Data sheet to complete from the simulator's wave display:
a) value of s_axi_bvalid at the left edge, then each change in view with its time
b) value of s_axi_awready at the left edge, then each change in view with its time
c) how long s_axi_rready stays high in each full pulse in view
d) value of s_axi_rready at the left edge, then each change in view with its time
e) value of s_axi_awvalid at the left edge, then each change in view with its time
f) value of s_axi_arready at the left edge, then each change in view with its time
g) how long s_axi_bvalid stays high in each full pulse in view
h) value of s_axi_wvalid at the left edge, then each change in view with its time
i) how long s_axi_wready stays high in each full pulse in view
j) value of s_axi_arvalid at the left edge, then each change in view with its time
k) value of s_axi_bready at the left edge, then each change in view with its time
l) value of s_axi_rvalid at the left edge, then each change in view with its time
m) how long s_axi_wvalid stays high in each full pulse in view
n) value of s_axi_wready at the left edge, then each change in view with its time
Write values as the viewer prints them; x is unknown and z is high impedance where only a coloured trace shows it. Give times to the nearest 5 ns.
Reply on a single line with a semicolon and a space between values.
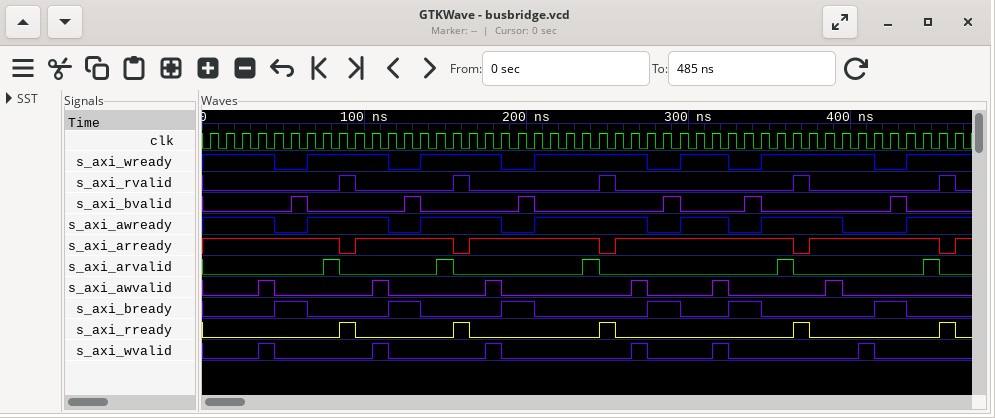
0, 1 at 55 ns, 0 at 65 ns, 1 at 125 ns, 0 at 135 ns, 1 at 195 ns, 0 at 205 ns, 1 at 285 ns, 0 at 295 ns, 1 at 335 ns, 0 at 345 ns, 1 at 425 ns, 0 at 435 ns; 1, 0 at 45 ns, 1 at 65 ns, 0 at 115 ns, 1 at 135 ns, 0 at 185 ns, 1 at 205 ns, 0 at 275 ns, 1 at 295 ns, 0 at 325 ns, 1 at 345 ns, 0 at 395 ns, 1 at 435 ns; 10 ns, 10 ns, 10 ns, 10 ns, 10 ns; 0, 1 at 85 ns, 0 at 95 ns, 1 at 155 ns, 0 at 165 ns, 1 at 245 ns, 0 at 255 ns, 1 at 365 ns, 0 at 375 ns, 1 at 455 ns, 0 at 465 ns; 0, 1 at 35 ns, 0 at 45 ns, 1 at 105 ns, 0 at 115 ns, 1 at 175 ns, 0 at 185 ns, 1 at 265 ns, 0 at 275 ns, 1 at 315 ns, 0 at 325 ns, 1 at 385 ns, 0 at 395 ns; 1, 0 at 85 ns, 1 at 95 ns, 0 at 155 ns, 1 at 165 ns, 0 at 245 ns, 1 at 255 ns, 0 at 365 ns, 1 at 375 ns, 0 at 455 ns, 1 at 465 ns; 10 ns, 10 ns, 10 ns, 10 ns, 10 ns, 10 ns; 0, 1 at 35 ns, 0 at 45 ns, 1 at 105 ns, 0 at 115 ns, 1 at 175 ns, 0 at 185 ns, 1 at 265 ns, 0 at 275 ns, 1 at 315 ns, 0 at 325 ns, 1 at 405 ns, 0 at 415 ns; 50 ns, 50 ns, 70 ns, 30 ns, 70 ns; 0, 1 at 75 ns, 0 at 85 ns, 1 at 145 ns, 0 at 155 ns, 1 at 235 ns, 0 at 245 ns, 1 at 355 ns, 0 at 365 ns, 1 at 445 ns, 0 at 455 ns; 0, 1 at 45 ns, 0 at 65 ns, 1 at 115 ns, 0 at 135 ns, 1 at 185 ns, 0 at 205 ns, 1 at 275 ns, 0 at 295 ns, 1 at 325 ns, 0 at 345 ns, 1 at 415 ns, 0 at 435 ns; 0, 1 at 85 ns, 0 at 95 ns, 1 at 155 ns, 0 at 165 ns, 1 at 245 ns, 0 at 255 ns, 1 at 365 ns, 0 at 375 ns, 1 at 455 ns, 0 at 465 ns; 10 ns, 10 ns, 10 ns, 10 ns, 10 ns, 10 ns; 1, 0 at 45 ns, 1 at 65 ns, 0 at 115 ns, 1 at 135 ns, 0 at 185 ns, 1 at 205 ns, 0 at 275 ns, 1 at 295 ns, 0 at 325 ns, 1 at 345 ns, 0 at 415 ns, 1 at 435 ns
